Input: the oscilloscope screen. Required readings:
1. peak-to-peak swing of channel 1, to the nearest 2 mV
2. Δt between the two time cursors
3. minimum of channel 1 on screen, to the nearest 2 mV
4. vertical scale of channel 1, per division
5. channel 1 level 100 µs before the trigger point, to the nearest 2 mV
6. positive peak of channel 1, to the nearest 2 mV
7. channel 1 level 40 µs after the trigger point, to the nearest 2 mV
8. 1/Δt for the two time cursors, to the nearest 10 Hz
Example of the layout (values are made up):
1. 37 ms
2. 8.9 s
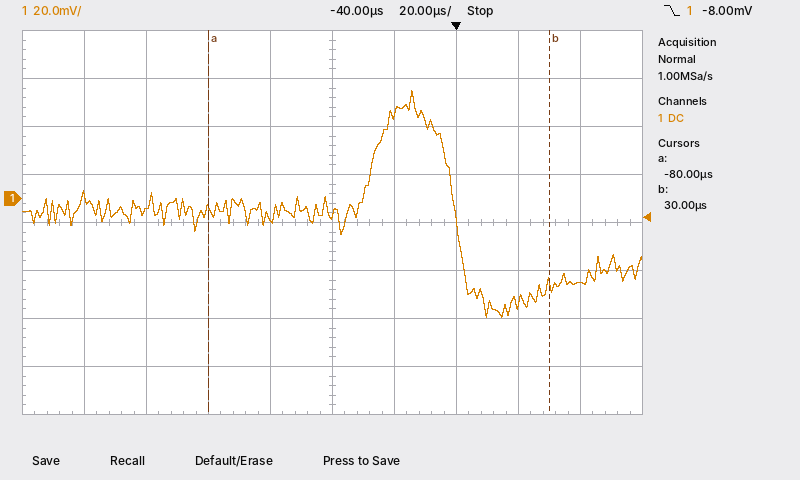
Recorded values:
1. 94 mV
2. 110 µs
3. -50 mV
4. 20 mV
5. -4 mV
6. 44 mV
7. -36 mV
8. 9.09 kHz
